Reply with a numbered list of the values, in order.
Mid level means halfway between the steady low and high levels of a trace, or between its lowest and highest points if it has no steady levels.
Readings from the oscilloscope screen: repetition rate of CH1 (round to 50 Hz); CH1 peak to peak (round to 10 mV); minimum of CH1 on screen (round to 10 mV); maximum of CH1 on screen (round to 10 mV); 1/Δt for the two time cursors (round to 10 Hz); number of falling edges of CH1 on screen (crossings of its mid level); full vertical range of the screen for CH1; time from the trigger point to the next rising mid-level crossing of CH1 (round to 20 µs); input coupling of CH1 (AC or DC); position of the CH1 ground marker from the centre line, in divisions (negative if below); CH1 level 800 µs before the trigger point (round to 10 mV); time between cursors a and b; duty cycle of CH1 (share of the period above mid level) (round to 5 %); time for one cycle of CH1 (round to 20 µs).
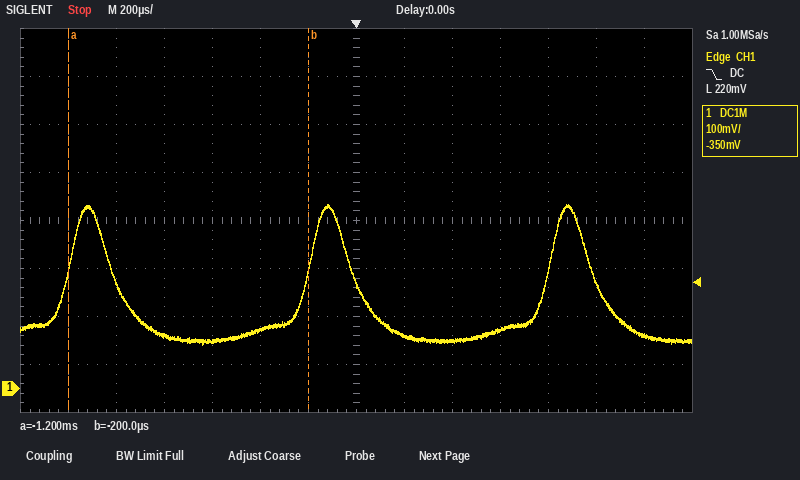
1. 1.00 kHz
2. 290 mV
3. 90 mV
4. 380 mV
5. 1.00 kHz
6. 3
7. 800 mV
8. 800 µs
9. DC
10. -3.5 div
11. 110 mV
12. 1.00 ms
13. 20 %
14. 1.00 ms
